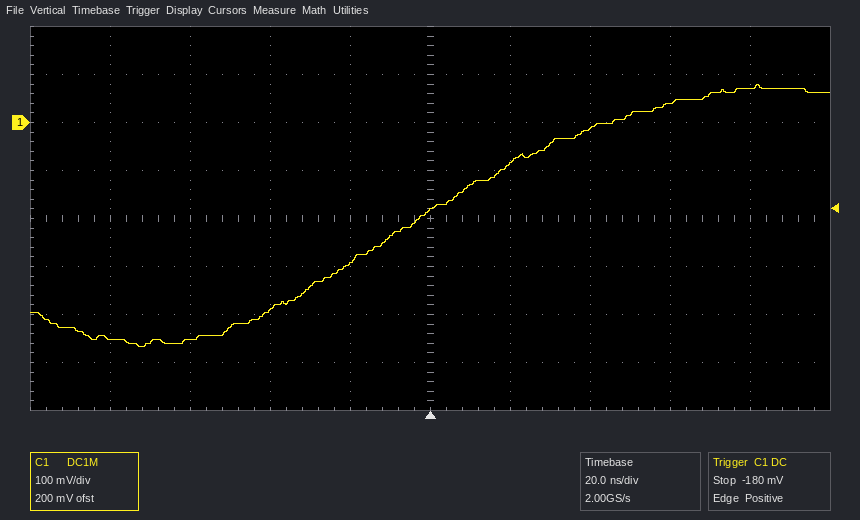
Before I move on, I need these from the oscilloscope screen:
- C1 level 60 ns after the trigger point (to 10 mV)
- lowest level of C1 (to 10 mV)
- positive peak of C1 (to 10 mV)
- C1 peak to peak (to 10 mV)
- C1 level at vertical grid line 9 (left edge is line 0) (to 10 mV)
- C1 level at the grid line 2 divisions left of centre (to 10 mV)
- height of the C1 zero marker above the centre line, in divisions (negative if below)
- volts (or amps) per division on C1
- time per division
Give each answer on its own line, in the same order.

40 mV
-470 mV
80 mV
550 mV
70 mV
-390 mV
+2.0 div
100 mV
20 ns
